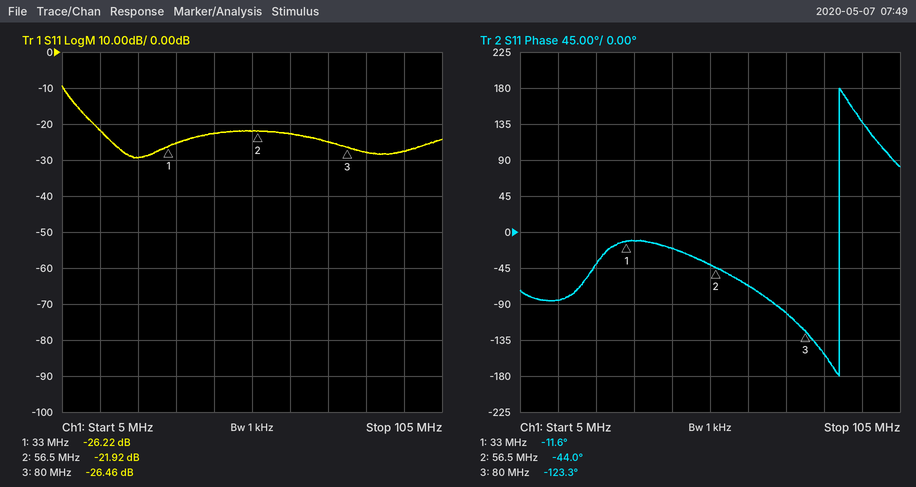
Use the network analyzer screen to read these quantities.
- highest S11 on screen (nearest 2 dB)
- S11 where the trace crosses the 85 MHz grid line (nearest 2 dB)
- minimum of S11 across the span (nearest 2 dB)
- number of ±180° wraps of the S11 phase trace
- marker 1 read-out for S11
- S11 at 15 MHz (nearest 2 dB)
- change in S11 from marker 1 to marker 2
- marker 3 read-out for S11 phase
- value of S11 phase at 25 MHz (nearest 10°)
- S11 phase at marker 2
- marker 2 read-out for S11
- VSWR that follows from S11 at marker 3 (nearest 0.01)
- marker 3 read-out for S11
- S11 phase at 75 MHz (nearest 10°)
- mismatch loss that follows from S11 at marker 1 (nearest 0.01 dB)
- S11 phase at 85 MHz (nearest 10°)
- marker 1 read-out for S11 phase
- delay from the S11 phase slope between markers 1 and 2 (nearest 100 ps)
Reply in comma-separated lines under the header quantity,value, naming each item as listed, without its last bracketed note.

quantity,value
highest S11 on screen,-10 dB
S11 where the trace crosses the 85 MHz grid line,-28 dB
minimum of S11 across the span,-30 dB
number of ±180° wraps of the S11 phase trace,1
marker 1 read-out for S11,-26.22 dB
S11 at 15 MHz,-22 dB
change in S11 from marker 1 to marker 2,4.30 dB
marker 3 read-out for S11 phase,-123.3°
value of S11 phase at 25 MHz,-40°
S11 phase at marker 2,-44.0°
marker 2 read-out for S11,-21.92 dB
VSWR that follows from S11 at marker 3,1.10
marker 3 read-out for S11,-26.46 dB
S11 phase at 75 MHz,-100°
mismatch loss that follows from S11 at marker 1,0.01 dB
S11 phase at 85 MHz,-150°
marker 1 read-out for S11 phase,-11.6°
delay from the S11 phase slope between markers 1 and 2,3.8 ns
